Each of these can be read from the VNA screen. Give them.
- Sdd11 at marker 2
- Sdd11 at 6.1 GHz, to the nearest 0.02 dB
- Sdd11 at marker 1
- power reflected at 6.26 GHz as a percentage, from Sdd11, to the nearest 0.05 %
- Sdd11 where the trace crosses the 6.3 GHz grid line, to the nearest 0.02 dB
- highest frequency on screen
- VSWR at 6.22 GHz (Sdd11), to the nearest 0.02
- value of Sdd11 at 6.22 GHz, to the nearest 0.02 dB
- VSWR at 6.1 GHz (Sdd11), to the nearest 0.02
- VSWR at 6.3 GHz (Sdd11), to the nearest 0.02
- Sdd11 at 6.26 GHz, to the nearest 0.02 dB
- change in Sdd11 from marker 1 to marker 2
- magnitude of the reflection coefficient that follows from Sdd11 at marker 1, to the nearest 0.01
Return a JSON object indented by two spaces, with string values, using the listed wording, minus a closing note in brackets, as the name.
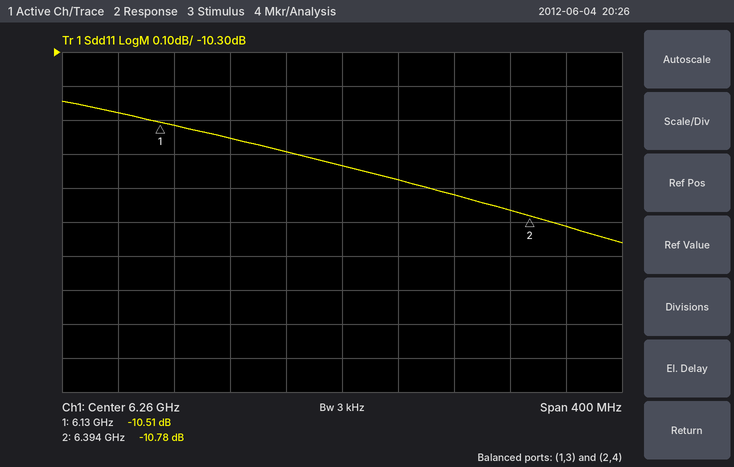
{
  "Sdd11 at marker 2": "-10.78 dB",
  "Sdd11 at 6.1 GHz, to the nearest 0.02 dB": "-10.48 dB",
  "Sdd11 at marker 1": "-10.51 dB",
  "power reflected at 6.26 GHz as a percentage, from Sdd11, to the nearest 0.05 %": "8.65 %",
  "Sdd11 where the trace crosses the 6.3 GHz grid line, to the nearest 0.02 dB": "-10.68 dB",
  "highest frequency on screen": "6.46 GHz",
  "VSWR at 6.22 GHz (Sdd11), to the nearest 0.02": "1.84",
  "value of Sdd11 at 6.22 GHz, to the nearest 0.02 dB": "-10.60 dB",
  "VSWR at 6.1 GHz (Sdd11), to the nearest 0.02": "1.86",
  "VSWR at 6.3 GHz (Sdd11), to the nearest 0.02": "1.82",
  "Sdd11 at 6.26 GHz, to the nearest 0.02 dB": "-10.64 dB",
  "change in Sdd11 from marker 1 to marker 2": "-0.27 dB",
  "magnitude of the reflection coefficient that follows from Sdd11 at marker 1, to the nearest 0.01": "0.30"
}
